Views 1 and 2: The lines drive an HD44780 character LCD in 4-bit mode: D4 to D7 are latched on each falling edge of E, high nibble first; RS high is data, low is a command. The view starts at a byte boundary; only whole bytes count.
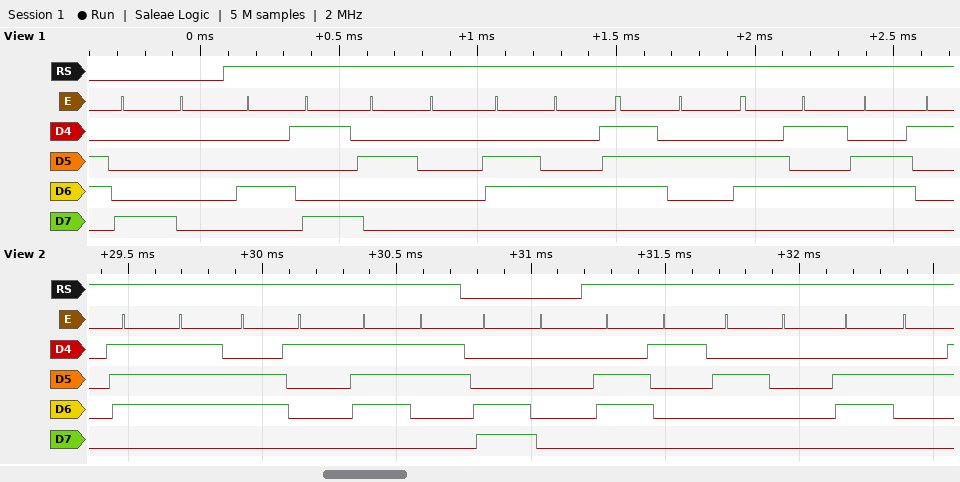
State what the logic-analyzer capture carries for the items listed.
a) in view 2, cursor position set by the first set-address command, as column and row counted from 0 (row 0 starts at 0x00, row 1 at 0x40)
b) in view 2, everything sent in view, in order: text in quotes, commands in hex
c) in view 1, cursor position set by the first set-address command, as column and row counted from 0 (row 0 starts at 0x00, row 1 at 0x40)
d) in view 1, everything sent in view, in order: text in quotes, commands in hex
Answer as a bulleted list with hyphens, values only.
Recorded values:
- column 0, row 1
- "was" 0xC0 "a b"
- column 0, row 0
- 0x80 "I drea"
